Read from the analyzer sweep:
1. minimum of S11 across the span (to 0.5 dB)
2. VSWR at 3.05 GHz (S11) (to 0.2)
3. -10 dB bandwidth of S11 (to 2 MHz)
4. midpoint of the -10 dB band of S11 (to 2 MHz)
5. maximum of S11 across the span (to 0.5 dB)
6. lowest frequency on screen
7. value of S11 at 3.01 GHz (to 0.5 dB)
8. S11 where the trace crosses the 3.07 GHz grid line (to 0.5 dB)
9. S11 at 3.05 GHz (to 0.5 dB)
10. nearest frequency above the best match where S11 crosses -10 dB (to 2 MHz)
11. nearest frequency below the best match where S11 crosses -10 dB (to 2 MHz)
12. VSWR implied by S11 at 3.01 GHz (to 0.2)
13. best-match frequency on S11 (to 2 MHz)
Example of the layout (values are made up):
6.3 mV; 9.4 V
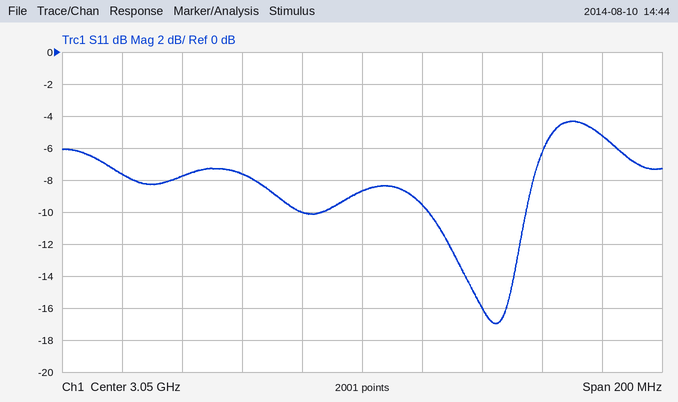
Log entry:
-17.0 dB; 2.2; 32 MHz; 3.088 GHz; -4.5 dB; 2.95 GHz; -7.5 dB; -9.5 dB; -8.5 dB; 3.104 GHz; 3.072 GHz; 2.4; 3.094 GHz
